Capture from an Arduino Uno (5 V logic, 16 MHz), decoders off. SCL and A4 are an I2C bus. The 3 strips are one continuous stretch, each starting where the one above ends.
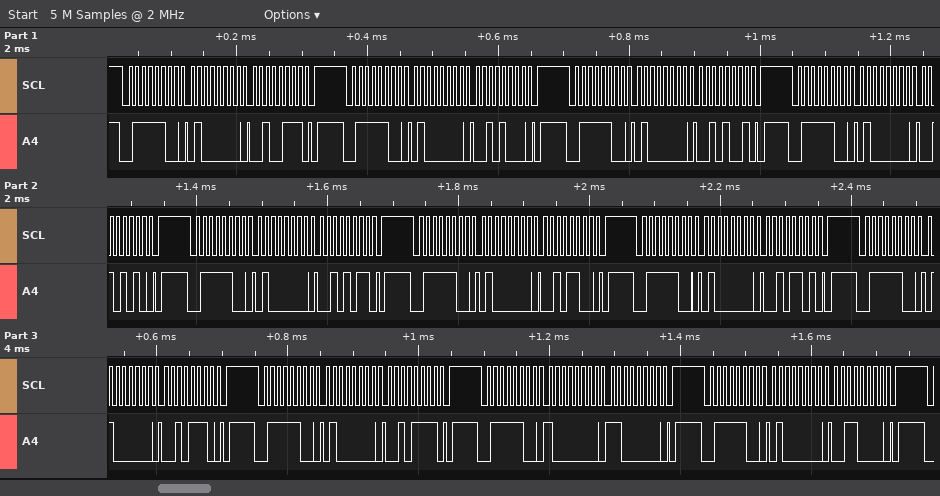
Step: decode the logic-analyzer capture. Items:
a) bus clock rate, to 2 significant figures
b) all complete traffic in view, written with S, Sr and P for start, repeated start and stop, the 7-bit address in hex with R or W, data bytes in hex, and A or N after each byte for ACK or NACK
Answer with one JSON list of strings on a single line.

["100 kHz", "S 3EW A 40 A 27 A P S 3EW A 40 A 28 A P S 3EW A 40 A 29 A P S 3EW A 40 A 2A A P S 3EW A 40 A 2B A P S 3EW A 40 A 2C A P S 3EW A 40 A 2D A P S 3EW A 40 A 2E A P S 3EW A 40 A 2F A P S 3EW A 80 A C0 A P S 3EW A 40 A 30 A P"]
